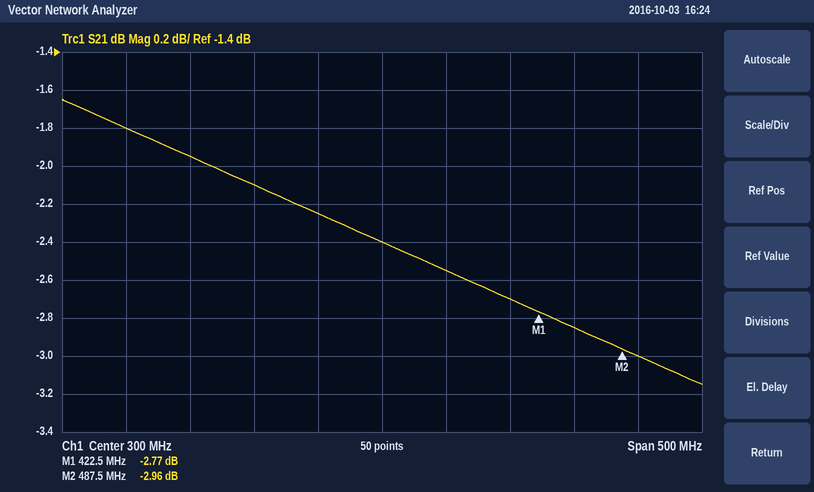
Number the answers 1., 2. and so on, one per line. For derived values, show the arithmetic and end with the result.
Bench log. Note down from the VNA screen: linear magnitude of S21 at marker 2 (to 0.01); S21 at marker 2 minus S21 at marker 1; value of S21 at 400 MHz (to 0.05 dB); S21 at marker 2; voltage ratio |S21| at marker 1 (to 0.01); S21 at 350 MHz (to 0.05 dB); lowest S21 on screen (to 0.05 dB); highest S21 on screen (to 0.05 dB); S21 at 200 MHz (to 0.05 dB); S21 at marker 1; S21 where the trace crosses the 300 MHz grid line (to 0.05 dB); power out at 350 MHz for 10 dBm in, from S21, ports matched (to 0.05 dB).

1. 10^(-2.96/20) ≈ 0.71
2. -2.96 − (-2.77) = -0.19 dB
3. -2.70 dB
4. -2.96 dB
5. 10^(-2.77/20) ≈ 0.73
6. -2.55 dB
7. -3.15 dB
8. -1.65 dB
9. -2.10 dB
10. -2.77 dB
11. -2.40 dB
12. 10 dBm + (-2.55 dB) = 7.45 dBm
